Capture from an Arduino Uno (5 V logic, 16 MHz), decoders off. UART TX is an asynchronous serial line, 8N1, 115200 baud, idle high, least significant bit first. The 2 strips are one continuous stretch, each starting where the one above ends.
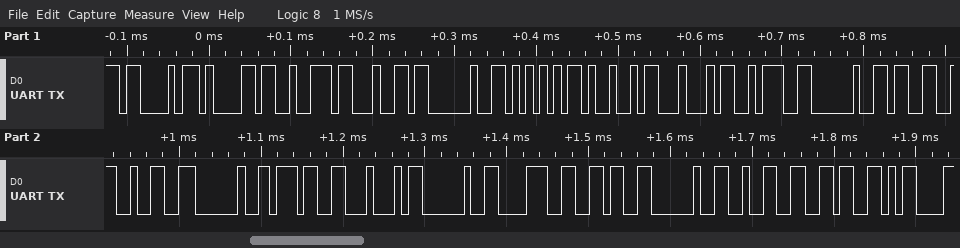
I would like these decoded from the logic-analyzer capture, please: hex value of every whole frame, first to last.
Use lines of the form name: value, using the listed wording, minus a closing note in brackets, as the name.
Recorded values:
hex value of every whole frame, first to last: 43 61 72 64 20 55 49 44 3A 20 33 32 20 37 44 20 38 36 20 32 36 0D
